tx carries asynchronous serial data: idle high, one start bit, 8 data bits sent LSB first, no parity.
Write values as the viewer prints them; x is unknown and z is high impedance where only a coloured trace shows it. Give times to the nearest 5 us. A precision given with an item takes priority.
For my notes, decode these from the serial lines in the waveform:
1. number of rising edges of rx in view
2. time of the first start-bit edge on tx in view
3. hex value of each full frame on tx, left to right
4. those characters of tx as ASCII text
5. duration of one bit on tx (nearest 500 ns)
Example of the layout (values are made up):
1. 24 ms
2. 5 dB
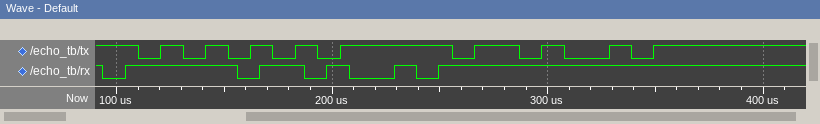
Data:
1. 5
2. 110 us
3. 55, 4B
4. "UK"
5. 10500 ns
